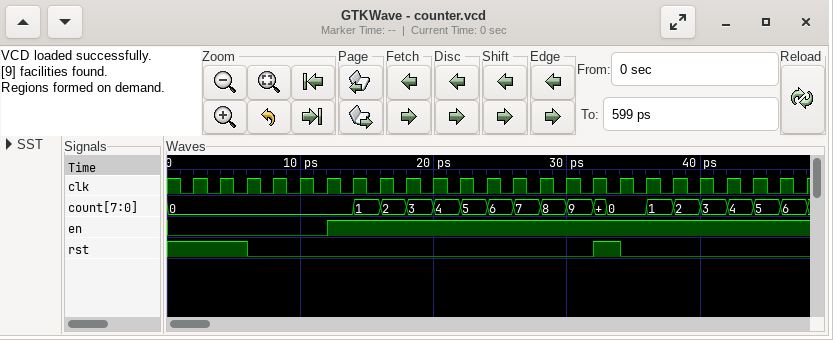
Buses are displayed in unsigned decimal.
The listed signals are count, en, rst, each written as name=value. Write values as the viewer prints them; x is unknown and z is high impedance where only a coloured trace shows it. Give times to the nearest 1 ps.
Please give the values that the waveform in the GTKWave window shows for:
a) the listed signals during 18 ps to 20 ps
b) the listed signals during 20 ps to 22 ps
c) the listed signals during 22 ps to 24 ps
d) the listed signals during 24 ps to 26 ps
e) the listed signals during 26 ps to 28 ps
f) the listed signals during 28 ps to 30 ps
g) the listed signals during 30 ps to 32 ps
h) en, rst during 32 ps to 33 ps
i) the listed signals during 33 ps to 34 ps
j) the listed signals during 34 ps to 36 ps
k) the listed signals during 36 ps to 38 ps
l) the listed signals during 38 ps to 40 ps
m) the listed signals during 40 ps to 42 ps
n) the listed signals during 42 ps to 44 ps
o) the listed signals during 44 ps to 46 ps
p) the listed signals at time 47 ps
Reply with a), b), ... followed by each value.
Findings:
a) count=3, en=1, rst=0
b) count=4, en=1, rst=0
c) count=5, en=1, rst=0
d) count=6, en=1, rst=0
e) count=7, en=1, rst=0
f) count=8, en=1, rst=0
g) count=9, en=1, rst=0
h) en=1, rst=1
i) count=0, en=1, rst=1
j) count=0, en=1, rst=0
k) count=1, en=1, rst=0
l) count=2, en=1, rst=0
m) count=3, en=1, rst=0
n) count=4, en=1, rst=0
o) count=5, en=1, rst=0
p) count=6, en=1, rst=0
